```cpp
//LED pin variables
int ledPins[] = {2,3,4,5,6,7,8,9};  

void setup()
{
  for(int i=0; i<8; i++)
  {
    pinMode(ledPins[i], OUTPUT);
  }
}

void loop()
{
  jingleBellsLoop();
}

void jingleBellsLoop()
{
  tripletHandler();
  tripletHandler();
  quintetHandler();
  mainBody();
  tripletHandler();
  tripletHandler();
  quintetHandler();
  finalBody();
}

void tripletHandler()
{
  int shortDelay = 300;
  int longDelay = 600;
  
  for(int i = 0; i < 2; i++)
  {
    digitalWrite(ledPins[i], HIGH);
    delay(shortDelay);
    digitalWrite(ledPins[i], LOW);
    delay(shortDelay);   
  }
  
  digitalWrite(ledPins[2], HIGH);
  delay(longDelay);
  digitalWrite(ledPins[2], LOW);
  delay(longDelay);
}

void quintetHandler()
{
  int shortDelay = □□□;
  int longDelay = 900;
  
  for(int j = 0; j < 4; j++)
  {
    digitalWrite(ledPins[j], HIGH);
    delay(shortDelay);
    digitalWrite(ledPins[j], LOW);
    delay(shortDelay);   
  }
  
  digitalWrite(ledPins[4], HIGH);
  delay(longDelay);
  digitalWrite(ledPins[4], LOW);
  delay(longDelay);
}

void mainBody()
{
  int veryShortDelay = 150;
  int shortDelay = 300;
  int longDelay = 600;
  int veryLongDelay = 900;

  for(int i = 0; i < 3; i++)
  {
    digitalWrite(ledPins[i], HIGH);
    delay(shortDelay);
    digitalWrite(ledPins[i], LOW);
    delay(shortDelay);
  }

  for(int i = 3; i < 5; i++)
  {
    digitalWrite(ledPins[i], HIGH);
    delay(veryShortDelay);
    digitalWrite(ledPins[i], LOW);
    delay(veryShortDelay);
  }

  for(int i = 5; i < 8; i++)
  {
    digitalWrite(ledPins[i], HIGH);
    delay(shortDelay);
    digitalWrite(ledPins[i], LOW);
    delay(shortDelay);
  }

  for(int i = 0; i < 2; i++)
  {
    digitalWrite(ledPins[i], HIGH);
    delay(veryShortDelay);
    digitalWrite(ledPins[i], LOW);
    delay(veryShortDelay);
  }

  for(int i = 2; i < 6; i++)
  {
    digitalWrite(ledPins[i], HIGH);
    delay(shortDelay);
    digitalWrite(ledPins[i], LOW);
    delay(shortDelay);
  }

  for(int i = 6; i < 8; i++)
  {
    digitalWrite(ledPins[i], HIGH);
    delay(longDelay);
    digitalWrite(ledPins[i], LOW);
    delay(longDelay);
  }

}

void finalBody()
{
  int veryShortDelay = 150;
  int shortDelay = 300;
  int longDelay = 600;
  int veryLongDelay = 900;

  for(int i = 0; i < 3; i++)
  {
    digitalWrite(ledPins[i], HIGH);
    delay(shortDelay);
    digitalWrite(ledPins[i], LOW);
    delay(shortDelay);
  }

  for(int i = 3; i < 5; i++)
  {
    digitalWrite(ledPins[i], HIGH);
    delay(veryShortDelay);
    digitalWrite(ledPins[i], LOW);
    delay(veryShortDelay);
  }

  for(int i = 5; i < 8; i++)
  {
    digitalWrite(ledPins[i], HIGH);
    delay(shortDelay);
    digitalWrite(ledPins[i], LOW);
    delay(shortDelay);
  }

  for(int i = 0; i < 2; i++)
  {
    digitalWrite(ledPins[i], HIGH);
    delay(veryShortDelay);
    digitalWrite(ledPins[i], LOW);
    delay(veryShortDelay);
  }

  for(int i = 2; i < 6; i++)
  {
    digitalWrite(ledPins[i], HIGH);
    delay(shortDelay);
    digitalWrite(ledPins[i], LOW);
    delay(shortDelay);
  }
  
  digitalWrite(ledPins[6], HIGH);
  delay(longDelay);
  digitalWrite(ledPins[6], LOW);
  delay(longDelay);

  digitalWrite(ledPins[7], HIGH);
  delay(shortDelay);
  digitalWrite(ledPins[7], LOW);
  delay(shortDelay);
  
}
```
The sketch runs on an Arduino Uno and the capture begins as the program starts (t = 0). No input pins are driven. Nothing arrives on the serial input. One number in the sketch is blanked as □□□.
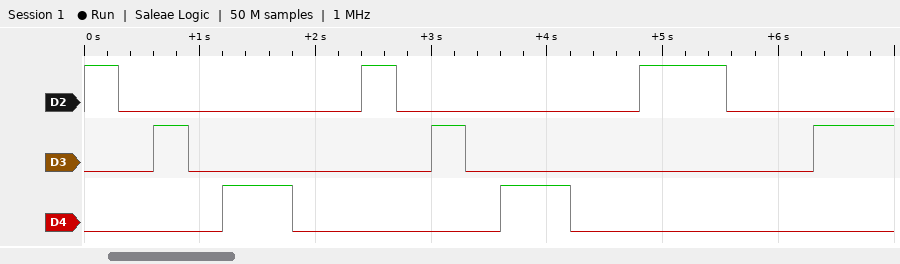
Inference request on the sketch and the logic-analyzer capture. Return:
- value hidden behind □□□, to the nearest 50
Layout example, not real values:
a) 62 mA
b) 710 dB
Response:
a) 750
